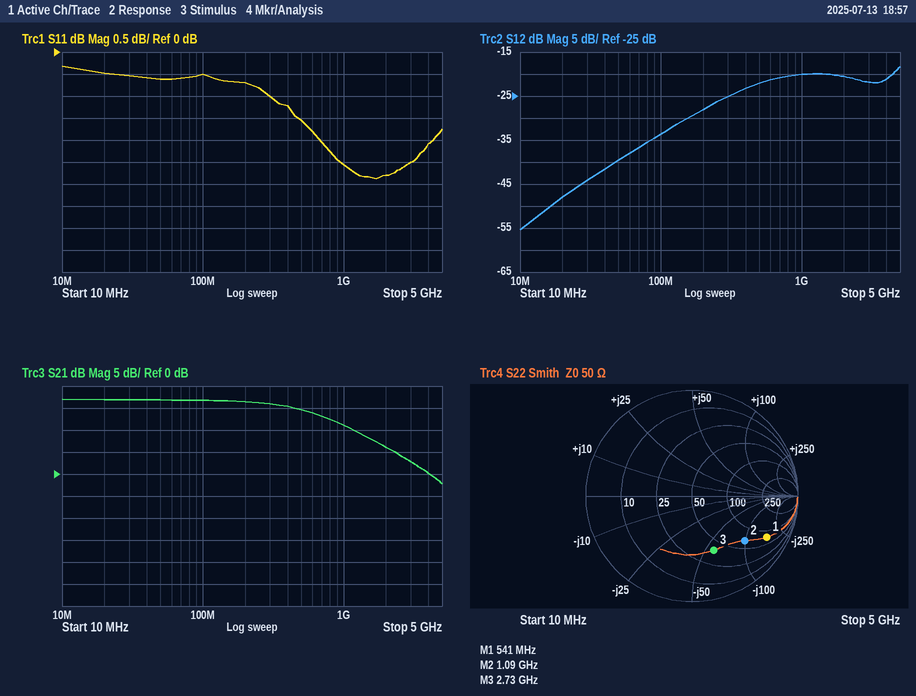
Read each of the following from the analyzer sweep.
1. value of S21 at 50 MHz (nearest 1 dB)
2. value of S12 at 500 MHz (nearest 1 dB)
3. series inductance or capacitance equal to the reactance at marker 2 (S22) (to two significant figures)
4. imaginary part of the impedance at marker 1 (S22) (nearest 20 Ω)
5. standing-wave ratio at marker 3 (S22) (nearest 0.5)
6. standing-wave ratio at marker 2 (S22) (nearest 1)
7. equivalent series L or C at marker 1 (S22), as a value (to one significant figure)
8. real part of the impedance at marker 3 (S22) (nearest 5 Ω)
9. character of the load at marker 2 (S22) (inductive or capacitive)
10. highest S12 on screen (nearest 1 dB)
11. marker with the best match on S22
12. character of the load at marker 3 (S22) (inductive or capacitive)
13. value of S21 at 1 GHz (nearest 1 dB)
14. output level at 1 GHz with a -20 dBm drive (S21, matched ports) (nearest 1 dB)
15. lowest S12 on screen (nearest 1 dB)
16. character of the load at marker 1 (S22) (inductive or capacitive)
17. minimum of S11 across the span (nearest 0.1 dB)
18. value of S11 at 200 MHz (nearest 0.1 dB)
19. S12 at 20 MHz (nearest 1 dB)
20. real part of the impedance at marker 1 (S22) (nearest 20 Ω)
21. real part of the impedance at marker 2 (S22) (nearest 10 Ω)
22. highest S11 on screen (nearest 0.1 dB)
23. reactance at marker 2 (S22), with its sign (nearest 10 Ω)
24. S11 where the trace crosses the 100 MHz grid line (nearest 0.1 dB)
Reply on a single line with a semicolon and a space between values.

17 dB; -22 dB; 1.5 pF; -160 Ω; 3.5; 5; 2 pF; 40 Ω; capacitive; -18 dB; marker 3; capacitive; 11 dB; -9 dBm; -55 dB; capacitive; -2.9 dB; -0.7 dB; -48 dB; 80 Ω; 70 Ω; -0.3 dB; -100 Ω; -0.5 dB
